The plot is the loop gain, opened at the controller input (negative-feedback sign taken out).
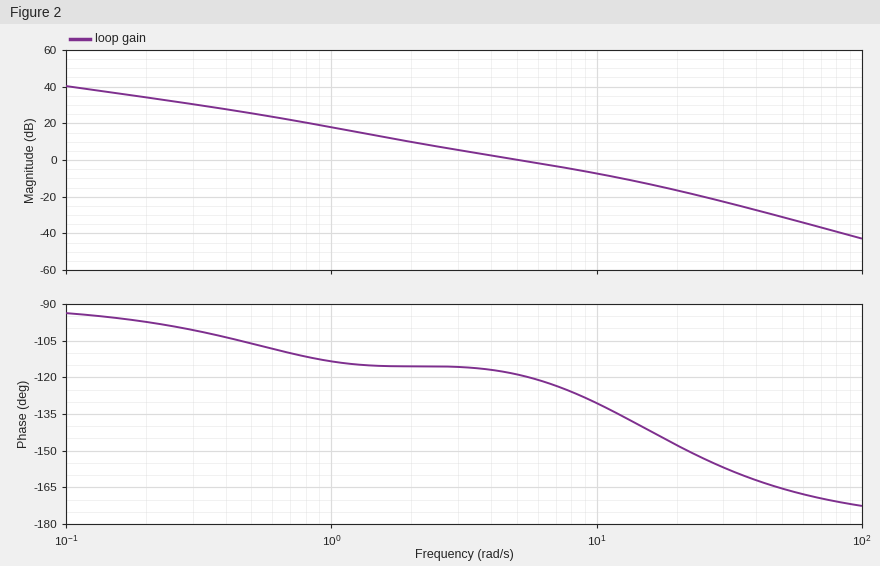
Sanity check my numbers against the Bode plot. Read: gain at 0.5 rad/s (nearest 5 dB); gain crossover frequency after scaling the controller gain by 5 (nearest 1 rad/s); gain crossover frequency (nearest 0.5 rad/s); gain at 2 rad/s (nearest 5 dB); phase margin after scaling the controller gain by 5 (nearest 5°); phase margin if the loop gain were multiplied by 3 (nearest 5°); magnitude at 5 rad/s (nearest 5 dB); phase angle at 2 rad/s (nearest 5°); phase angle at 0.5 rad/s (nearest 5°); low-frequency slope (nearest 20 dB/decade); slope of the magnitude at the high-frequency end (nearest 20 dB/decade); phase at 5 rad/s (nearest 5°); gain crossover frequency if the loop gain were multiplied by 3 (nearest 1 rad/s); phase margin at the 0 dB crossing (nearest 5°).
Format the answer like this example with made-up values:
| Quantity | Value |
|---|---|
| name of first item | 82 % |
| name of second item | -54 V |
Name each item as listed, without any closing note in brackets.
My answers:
| Quantity | Value |
|---|---|
| gain at 0.5 rad/s | 25 dB |
| gain crossover frequency after scaling the controller gain by 5 | 17 rad/s |
| gain crossover frequency | 5.0 rad/s |
| gain at 2 rad/s | 10 dB |
| phase margin after scaling the controller gain by 5 | 35° |
| phase margin if the loop gain were multiplied by 3 | 45° |
| magnitude at 5 rad/s | 0 dB |
| phase angle at 2 rad/s | -115° |
| phase angle at 0.5 rad/s | -105° |
| low-frequency slope | -20 dB/decade |
| slope of the magnitude at the high-frequency end | -40 dB/decade |
| phase at 5 rad/s | -120° |
| gain crossover frequency if the loop gain were multiplied by 3 | 12 rad/s |
| phase margin at the 0 dB crossing | 60° |
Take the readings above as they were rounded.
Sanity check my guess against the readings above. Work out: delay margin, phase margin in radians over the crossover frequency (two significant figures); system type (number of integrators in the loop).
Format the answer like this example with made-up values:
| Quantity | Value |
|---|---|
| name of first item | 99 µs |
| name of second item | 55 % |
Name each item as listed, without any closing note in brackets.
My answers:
| Quantity | Value |
|---|---|
| delay margin, phase margin in radians over the crossover frequency | 0.21 s |
| system type | 1 |
